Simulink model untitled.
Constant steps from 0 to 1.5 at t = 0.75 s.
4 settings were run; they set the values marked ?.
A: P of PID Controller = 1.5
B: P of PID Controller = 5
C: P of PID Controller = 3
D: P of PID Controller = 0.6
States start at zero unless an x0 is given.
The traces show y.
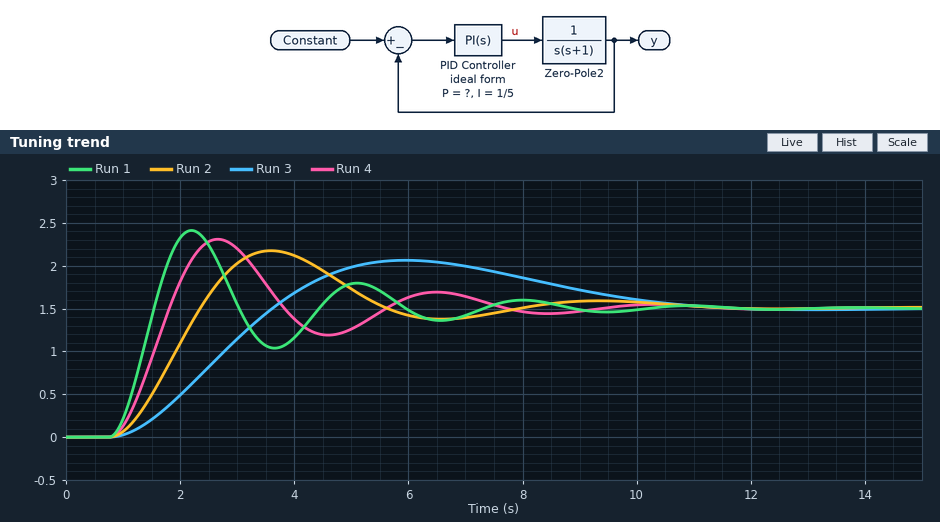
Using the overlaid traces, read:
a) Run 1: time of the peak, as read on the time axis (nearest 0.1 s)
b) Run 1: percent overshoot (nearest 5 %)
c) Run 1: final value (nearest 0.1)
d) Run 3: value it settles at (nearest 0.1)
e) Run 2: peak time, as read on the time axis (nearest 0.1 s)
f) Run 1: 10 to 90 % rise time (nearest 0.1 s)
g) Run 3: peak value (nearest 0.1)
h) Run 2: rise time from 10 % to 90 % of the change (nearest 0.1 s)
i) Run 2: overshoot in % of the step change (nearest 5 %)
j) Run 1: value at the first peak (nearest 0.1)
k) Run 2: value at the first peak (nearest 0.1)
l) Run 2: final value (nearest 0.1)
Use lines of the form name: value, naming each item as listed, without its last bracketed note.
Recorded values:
Run 1: time of the peak, as read on the time axis: 2.2 s
Run 1: percent overshoot: 60 %
Run 1: final value: 1.5
Run 3: value it settles at: 1.5
Run 2: peak time, as read on the time axis: 3.6 s
Run 1: 10 to 90 % rise time: 0.5 s
Run 3: peak value: 2.1
Run 2: rise time from 10 % to 90 % of the change: 1.1 s
Run 2: overshoot in % of the step change: 45 %
Run 1: value at the first peak: 2.4
Run 2: value at the first peak: 2.2
Run 2: final value: 1.5
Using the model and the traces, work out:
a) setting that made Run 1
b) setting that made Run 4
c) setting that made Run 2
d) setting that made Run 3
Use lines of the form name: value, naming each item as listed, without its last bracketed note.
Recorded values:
setting that made Run 1: B
setting that made Run 4: C
setting that made Run 2: A
setting that made Run 3: D
